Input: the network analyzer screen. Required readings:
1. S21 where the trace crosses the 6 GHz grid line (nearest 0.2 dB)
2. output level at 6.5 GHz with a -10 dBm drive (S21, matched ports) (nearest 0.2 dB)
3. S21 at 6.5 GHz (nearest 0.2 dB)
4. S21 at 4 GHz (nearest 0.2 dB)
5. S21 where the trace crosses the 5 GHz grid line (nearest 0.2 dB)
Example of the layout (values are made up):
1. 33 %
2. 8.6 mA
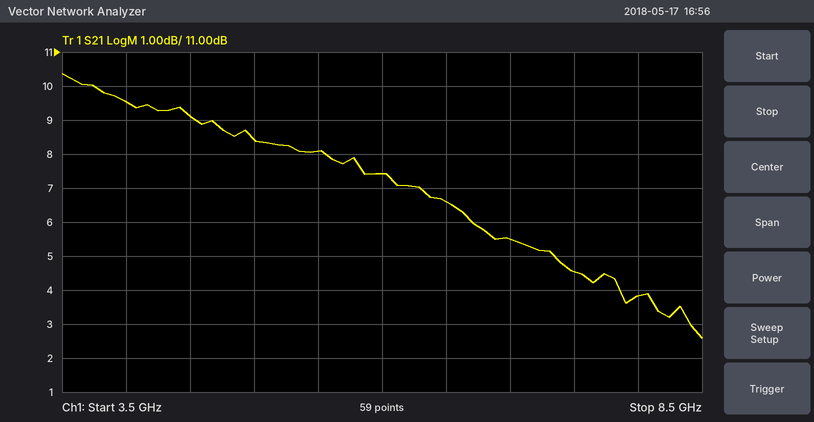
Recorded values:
1. 7.4 dB
2. -3.4 dBm
3. 6.6 dB
4. 9.6 dB
5. 8.4 dB
